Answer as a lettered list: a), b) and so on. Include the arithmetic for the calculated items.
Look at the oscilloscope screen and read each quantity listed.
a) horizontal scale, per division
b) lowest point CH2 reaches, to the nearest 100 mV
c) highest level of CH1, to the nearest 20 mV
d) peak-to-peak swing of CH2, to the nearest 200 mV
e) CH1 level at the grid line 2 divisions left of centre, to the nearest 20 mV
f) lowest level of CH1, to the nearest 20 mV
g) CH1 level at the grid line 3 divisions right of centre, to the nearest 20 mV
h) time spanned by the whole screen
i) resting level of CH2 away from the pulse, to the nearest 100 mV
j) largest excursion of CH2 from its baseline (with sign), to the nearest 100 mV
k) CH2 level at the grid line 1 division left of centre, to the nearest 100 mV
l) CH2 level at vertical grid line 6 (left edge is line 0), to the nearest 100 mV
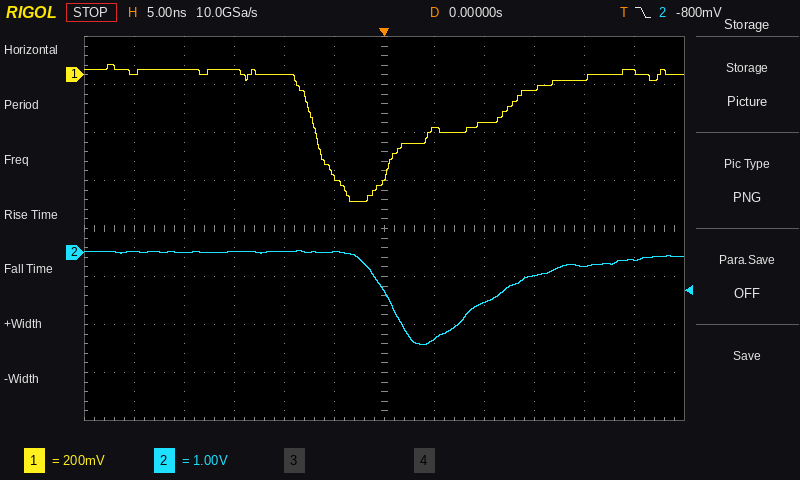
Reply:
a) 5 ns
b) -1.9 V
c) 40 mV
d) 2.0 V
e) 0 mV
f) -520 mV
g) -60 mV
h) 60 ns
i) 0.0 V
j) -1.9 V − (0.0 V) = -1.9 V
k) 0.0 V
l) -800 mV
